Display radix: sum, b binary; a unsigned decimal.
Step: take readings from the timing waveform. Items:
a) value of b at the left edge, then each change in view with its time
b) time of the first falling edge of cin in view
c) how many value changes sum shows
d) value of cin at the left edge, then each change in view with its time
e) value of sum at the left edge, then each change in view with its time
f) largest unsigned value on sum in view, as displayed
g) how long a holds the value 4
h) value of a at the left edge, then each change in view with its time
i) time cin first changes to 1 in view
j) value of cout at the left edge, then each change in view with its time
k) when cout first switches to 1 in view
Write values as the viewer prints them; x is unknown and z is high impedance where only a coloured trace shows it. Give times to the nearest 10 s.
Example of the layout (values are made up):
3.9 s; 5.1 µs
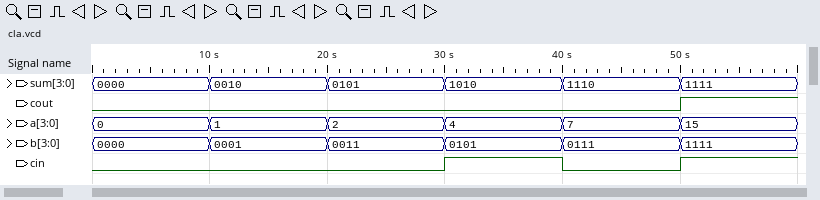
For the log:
0000, 0001 at 10 s, 0011 at 20 s, 0101 at 30 s, 0111 at 40 s, 1111 at 50 s; 40 s; 5; 0, 1 at 30 s, 0 at 40 s, 1 at 50 s; 0000, 0010 at 10 s, 0101 at 20 s, 1010 at 30 s, 1110 at 40 s, 1111 at 50 s; 1111; 10 s; 0, 1 at 10 s, 2 at 20 s, 4 at 30 s, 7 at 40 s, 15 at 50 s; 30 s; 0, 1 at 50 s; 50 s
